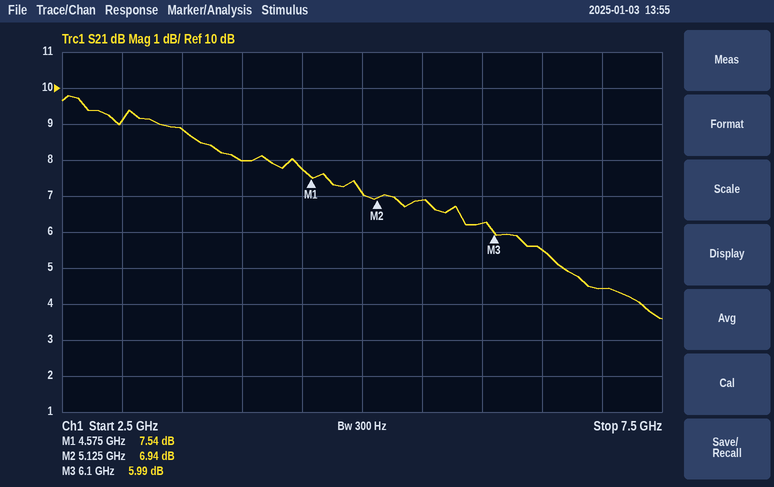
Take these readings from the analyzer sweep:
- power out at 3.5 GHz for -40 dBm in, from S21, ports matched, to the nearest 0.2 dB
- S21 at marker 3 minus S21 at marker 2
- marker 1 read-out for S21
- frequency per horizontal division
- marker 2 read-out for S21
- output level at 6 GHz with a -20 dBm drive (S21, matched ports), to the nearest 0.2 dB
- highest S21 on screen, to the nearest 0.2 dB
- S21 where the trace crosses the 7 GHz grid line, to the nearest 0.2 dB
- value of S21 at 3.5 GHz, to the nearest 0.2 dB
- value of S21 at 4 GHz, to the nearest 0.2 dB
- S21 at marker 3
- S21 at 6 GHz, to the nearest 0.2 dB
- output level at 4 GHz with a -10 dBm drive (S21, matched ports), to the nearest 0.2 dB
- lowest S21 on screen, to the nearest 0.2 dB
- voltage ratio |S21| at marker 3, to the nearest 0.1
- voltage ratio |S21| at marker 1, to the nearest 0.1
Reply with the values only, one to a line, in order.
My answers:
-31.2 dBm
-0.95 dB
7.54 dB
500 MHz
6.94 dB
-13.8 dBm
9.8 dB
4.4 dB
8.8 dB
8.0 dB
5.99 dB
6.2 dB
-2.0 dBm
3.6 dB
2.0
2.4
